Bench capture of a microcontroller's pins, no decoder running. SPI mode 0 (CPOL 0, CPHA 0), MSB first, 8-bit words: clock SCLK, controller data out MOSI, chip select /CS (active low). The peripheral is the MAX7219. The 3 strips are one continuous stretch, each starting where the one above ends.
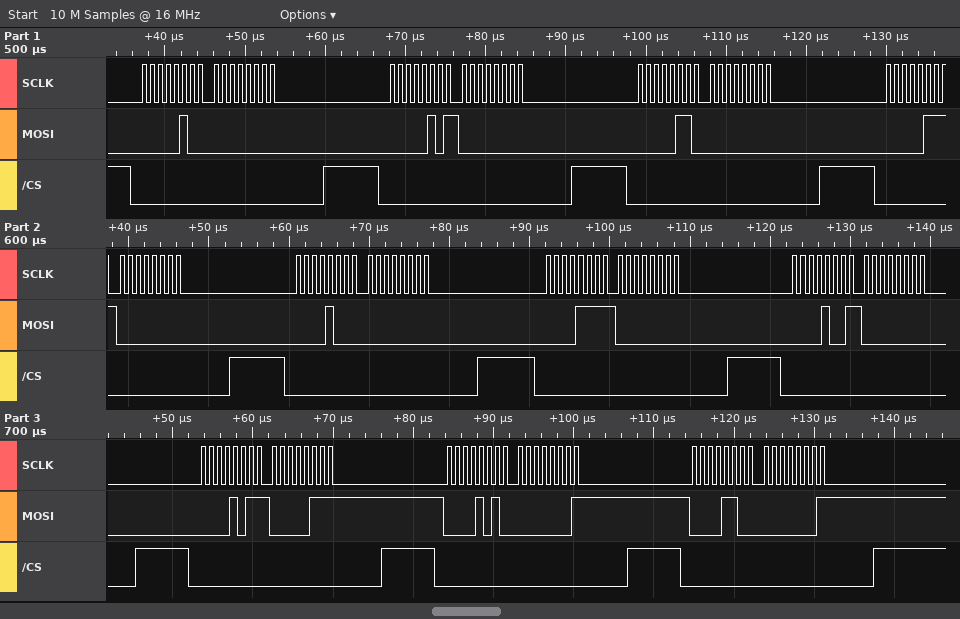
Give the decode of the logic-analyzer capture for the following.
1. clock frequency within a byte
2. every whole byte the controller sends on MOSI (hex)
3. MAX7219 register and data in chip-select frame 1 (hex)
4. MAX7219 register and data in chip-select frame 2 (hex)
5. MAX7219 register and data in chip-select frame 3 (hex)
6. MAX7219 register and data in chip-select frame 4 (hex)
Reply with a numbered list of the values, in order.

1. 1 MHz
2. 0x04 0x00 0x05 0x00 0x06 0x00 0x07 0x00 0x08 0x00 0x0F 0x00 0x09 0x00 0x0B 0x07 0x0A 0x01 0x0C 0x01
3. register 0x4, data 0x00
4. register 0x5, data 0x00
5. register 0x6, data 0x00
6. register 0x7, data 0x00
